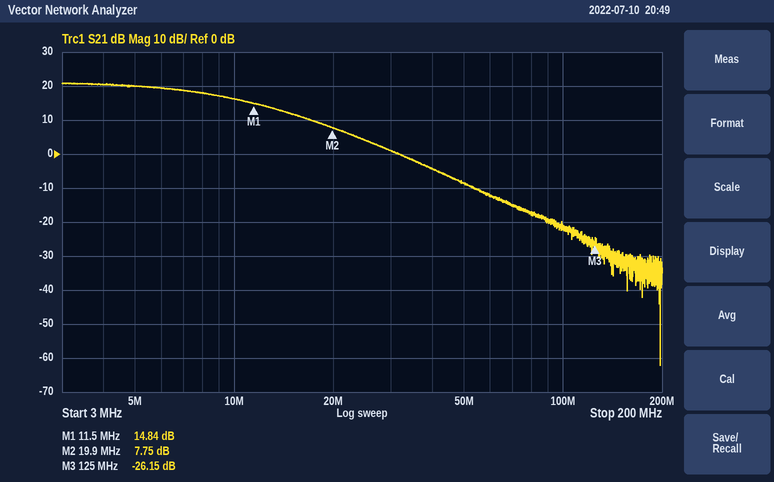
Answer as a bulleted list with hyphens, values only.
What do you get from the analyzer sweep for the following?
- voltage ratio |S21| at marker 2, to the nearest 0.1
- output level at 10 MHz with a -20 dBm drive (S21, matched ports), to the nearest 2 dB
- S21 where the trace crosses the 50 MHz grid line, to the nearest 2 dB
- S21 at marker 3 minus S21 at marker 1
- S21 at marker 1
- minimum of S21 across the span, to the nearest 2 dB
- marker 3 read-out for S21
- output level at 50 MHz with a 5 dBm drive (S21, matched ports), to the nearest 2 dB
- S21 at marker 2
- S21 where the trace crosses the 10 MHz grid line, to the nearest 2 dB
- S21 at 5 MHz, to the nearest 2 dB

- 2.4
- -4 dBm
- -8 dB
- -40.99 dB
- 14.84 dB
- -62 dB
- -26.15 dB
- -4 dBm
- 7.75 dB
- 16 dB
- 20 dB
